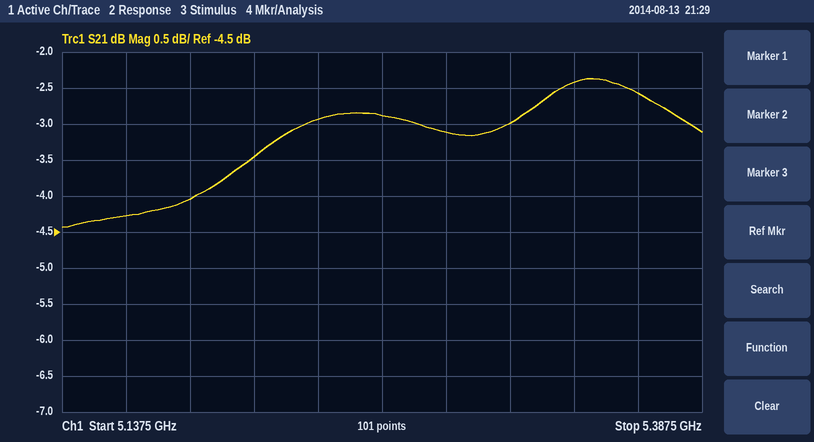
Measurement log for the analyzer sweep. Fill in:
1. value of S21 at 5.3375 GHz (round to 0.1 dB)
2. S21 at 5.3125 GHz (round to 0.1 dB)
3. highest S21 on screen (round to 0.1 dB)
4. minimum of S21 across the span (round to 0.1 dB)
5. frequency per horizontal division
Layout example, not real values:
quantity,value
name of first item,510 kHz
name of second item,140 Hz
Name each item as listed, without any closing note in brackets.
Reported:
quantity,value
value of S21 at 5.3375 GHz,-2.4 dB
S21 at 5.3125 GHz,-3.0 dB
highest S21 on screen,-2.4 dB
minimum of S21 across the span,-4.4 dB
frequency per horizontal division,25 MHz
